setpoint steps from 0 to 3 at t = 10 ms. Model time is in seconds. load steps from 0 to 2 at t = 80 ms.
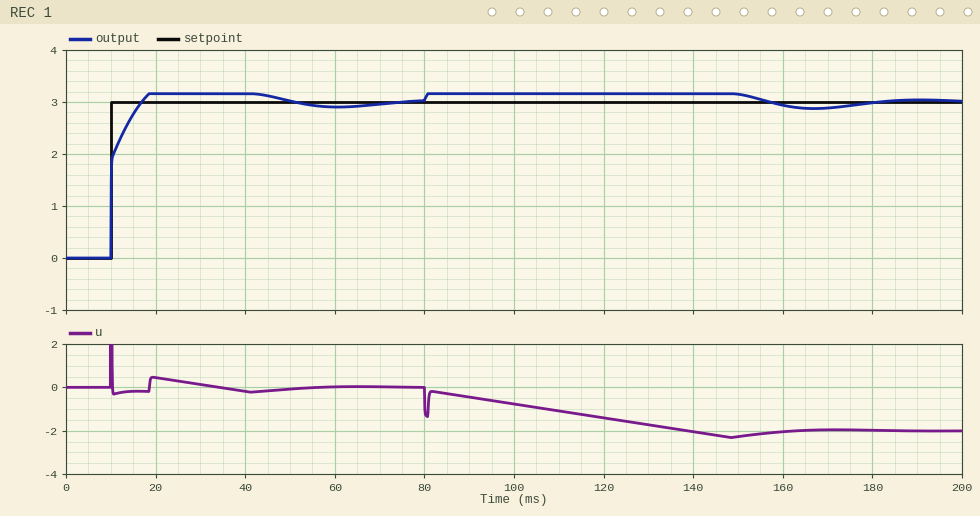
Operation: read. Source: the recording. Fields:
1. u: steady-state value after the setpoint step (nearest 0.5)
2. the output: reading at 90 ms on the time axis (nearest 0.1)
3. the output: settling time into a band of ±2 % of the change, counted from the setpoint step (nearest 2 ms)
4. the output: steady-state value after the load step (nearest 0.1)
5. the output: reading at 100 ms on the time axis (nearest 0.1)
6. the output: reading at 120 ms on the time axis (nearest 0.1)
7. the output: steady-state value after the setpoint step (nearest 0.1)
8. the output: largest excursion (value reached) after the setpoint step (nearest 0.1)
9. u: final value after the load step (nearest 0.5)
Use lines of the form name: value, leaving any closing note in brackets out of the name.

u: steady-state value after the setpoint step: 0.0
the output: reading at 90 ms on the time axis: 3.2
the output: settling time into a band of ±2 % of the change, counted from the setpoint step: 58 ms
the output: steady-state value after the load step: 3.0
the output: reading at 100 ms on the time axis: 3.2
the output: reading at 120 ms on the time axis: 3.2
the output: steady-state value after the setpoint step: 3.0
the output: largest excursion (value reached) after the setpoint step: 3.2
u: final value after the load step: -2.0
